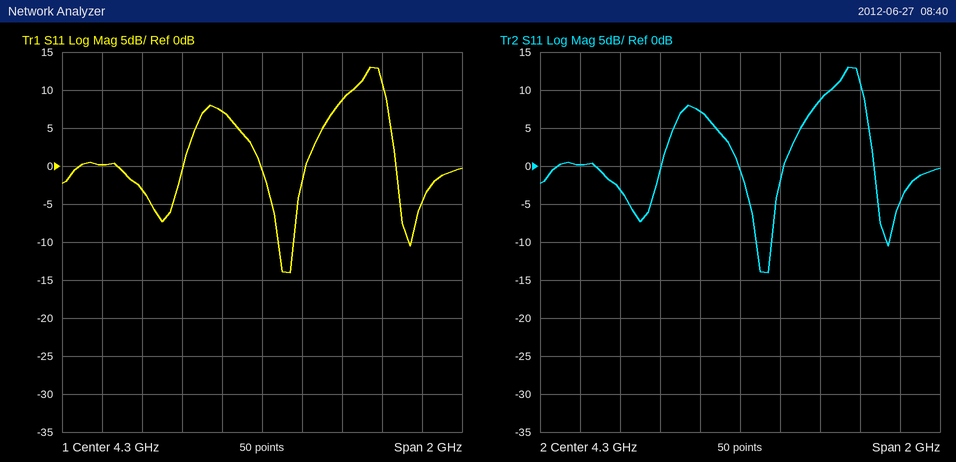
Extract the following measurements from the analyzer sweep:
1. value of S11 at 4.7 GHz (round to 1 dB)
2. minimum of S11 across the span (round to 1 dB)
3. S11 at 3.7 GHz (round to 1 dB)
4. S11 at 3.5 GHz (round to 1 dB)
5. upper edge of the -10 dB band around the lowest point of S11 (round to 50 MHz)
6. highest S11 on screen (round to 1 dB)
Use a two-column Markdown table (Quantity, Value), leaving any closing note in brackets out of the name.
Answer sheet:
| Quantity | Value |
|---|---|
| value of S11 at 4.7 GHz | 9 dB |
| minimum of S11 across the span | -14 dB |
| S11 at 3.7 GHz | -3 dB |
| S11 at 3.5 GHz | 0 dB |
| upper edge of the -10 dB band around the lowest point of S11 | 4.45 GHz |
| highest S11 on screen | 13 dB |
